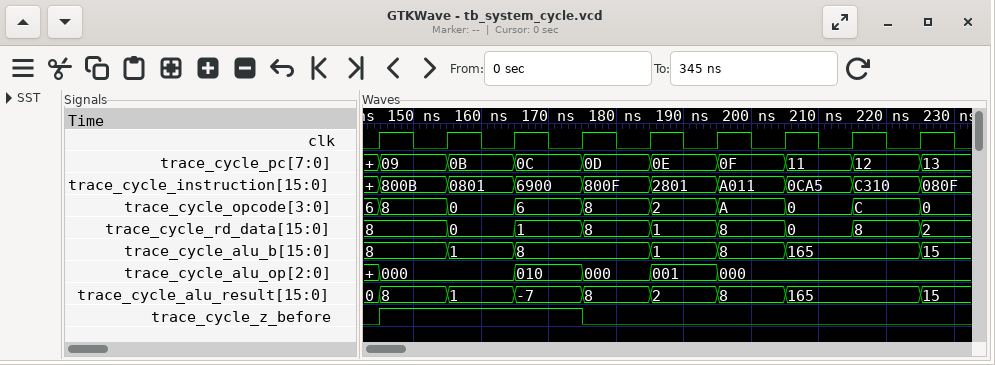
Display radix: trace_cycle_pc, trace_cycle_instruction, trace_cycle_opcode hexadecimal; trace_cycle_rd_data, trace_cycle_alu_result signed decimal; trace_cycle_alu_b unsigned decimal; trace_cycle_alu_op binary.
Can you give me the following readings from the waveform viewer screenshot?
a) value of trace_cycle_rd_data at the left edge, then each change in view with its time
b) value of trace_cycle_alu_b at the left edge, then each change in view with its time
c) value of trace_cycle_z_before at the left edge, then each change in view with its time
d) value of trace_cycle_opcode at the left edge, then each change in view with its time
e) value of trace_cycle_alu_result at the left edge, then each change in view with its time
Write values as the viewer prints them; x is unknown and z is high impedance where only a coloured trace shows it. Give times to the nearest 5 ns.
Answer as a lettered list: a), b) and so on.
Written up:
a) 8, 0 at 155 ns, 1 at 165 ns, 8 at 175 ns, 1 at 185 ns, 8 at 195 ns, 0 at 205 ns, 8 at 215 ns, 2 at 225 ns
b) 8, 1 at 155 ns, 8 at 165 ns, 1 at 185 ns, 8 at 195 ns, 165 at 205 ns, 15 at 225 ns
c) 0, 1 at 145 ns, 0 at 175 ns
d) 6, 8 at 145 ns, 0 at 155 ns, 6 at 165 ns, 8 at 175 ns, 2 at 185 ns, A at 195 ns, 0 at 205 ns, C at 215 ns, 0 at 225 ns
e) 0, 8 at 145 ns, 1 at 155 ns, -7 at 165 ns, 8 at 175 ns, 2 at 185 ns, 8 at 195 ns, 165 at 205 ns, 15 at 225 ns
